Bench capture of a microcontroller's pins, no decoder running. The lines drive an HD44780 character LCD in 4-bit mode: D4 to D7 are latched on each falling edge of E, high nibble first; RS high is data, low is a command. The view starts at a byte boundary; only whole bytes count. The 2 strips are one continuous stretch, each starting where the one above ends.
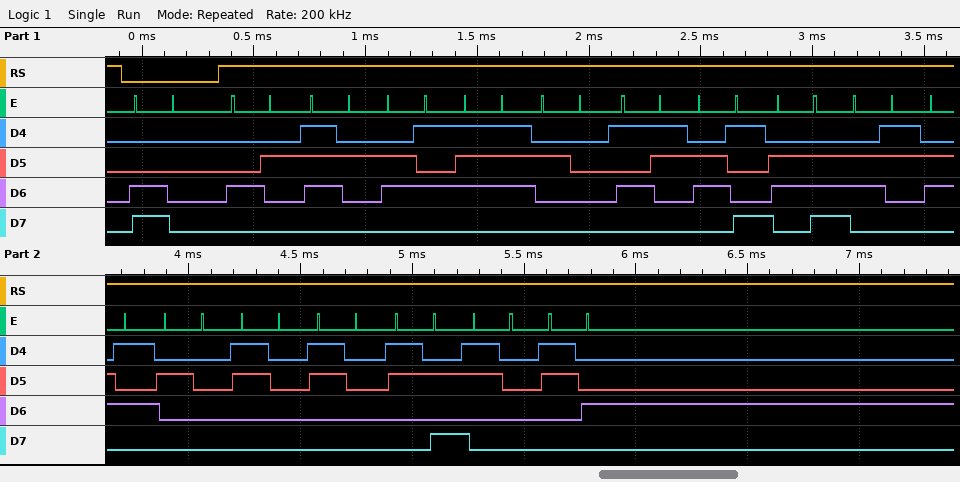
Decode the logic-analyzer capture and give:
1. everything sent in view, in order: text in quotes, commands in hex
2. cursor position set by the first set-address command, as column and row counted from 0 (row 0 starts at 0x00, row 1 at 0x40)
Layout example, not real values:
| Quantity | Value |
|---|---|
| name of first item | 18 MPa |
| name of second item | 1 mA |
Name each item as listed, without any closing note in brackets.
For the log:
| Quantity | Value |
|---|---|
| everything sent in view, in order: text in quotes, commands in hex | 0xC0 "Brew Since 00:04" |
| cursor position set by the first set-address command, as column and row counted from 0 | column 0, row 1 |
